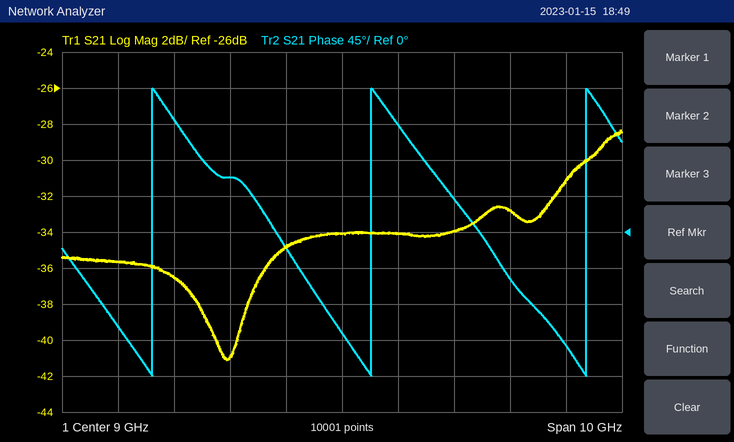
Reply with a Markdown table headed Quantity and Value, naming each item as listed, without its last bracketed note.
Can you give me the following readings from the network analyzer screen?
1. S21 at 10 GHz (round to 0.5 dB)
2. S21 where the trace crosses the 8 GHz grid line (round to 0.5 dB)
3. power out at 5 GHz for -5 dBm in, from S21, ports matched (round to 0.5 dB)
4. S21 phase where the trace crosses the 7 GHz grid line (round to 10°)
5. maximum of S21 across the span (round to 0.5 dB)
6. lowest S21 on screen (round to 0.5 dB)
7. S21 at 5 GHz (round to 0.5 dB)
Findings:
| Quantity | Value |
|---|---|
| S21 at 10 GHz | -34.0 dB |
| S21 where the trace crosses the 8 GHz grid line | -35.0 dB |
| power out at 5 GHz for -5 dBm in, from S21, ports matched | -40.5 dBm |
| S21 phase where the trace crosses the 7 GHz grid line | 70° |
| maximum of S21 across the span | -28.5 dB |
| lowest S21 on screen | -41.0 dB |
| S21 at 5 GHz | -35.5 dB |
